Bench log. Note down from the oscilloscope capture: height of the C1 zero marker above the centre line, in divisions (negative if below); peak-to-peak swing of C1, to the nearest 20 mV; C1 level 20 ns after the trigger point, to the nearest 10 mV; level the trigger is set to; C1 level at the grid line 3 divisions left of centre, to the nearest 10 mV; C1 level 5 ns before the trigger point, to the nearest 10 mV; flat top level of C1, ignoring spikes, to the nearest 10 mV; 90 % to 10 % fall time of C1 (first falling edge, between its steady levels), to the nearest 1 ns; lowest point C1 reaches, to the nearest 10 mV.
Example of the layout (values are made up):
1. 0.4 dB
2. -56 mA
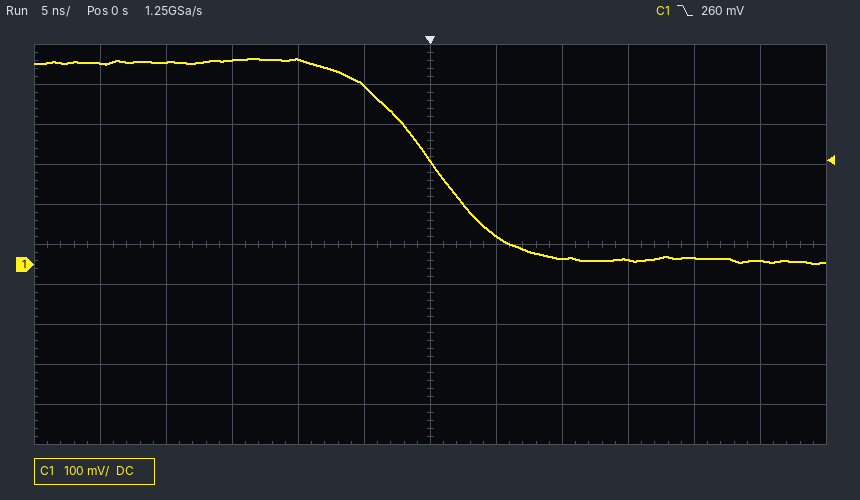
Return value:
1. -0.5 div
2. 520 mV
3. 20 mV
4. 260 mV
5. 510 mV
6. 450 mV
7. 510 mV
8. 11 ns
9. 0 mV
